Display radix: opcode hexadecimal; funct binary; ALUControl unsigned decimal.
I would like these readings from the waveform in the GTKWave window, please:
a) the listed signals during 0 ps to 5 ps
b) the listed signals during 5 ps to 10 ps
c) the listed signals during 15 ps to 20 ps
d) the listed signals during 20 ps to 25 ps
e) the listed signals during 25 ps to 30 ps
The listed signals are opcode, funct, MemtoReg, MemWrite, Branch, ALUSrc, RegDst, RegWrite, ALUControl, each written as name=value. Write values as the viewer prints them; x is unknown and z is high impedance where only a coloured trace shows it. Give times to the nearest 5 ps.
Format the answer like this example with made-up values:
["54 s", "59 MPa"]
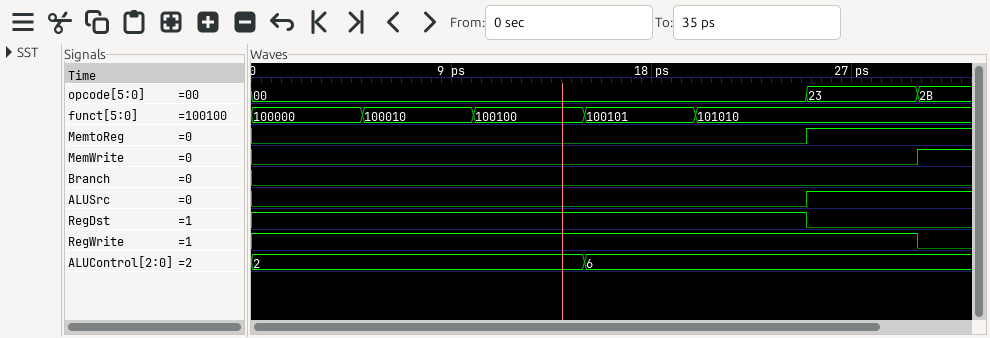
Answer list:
["opcode=00, funct=100000, MemtoReg=0, MemWrite=0, Branch=0, ALUSrc=0, RegDst=1, RegWrite=1, ALUControl=2", "opcode=00, funct=100010, MemtoReg=0, MemWrite=0, Branch=0, ALUSrc=0, RegDst=1, RegWrite=1, ALUControl=2", "opcode=00, funct=100101, MemtoReg=0, MemWrite=0, Branch=0, ALUSrc=0, RegDst=1, RegWrite=1, ALUControl=6", "opcode=00, funct=101010, MemtoReg=0, MemWrite=0, Branch=0, ALUSrc=0, RegDst=1, RegWrite=1, ALUControl=6", "opcode=23, funct=101010, MemtoReg=1, MemWrite=0, Branch=0, ALUSrc=1, RegDst=0, RegWrite=1, ALUControl=6"]
